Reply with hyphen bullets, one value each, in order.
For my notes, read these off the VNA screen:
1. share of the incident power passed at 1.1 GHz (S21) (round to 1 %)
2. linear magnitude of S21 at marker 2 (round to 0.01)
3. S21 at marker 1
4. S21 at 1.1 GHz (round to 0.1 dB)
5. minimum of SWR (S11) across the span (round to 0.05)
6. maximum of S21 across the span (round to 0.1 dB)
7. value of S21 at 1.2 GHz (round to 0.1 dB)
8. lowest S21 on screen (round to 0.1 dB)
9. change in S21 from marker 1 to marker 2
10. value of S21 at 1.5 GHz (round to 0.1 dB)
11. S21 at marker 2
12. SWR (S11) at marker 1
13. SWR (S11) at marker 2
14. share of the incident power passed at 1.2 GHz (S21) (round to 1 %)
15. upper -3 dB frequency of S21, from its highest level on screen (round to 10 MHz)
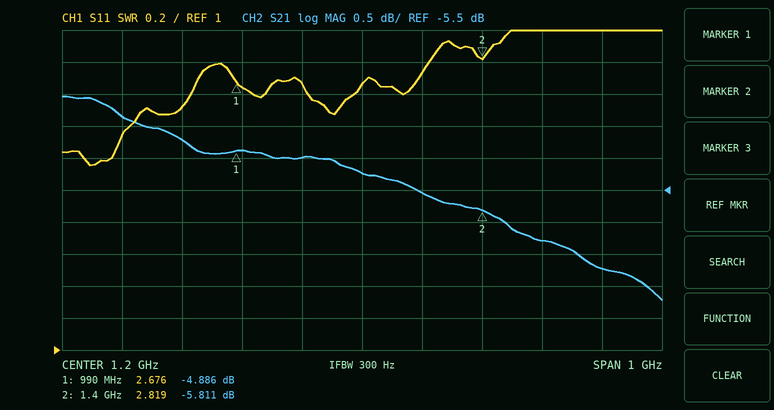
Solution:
- 32 %
- 0.51
- -4.886 dB
- -5.0 dB
- 2.15
- -4.0 dB
- -5.2 dB
- -7.2 dB
- -0.925 dB
- -6.3 dB
- -5.811 dB
- 2.676
- 2.819
- 30 %
- 1.68 GHz
